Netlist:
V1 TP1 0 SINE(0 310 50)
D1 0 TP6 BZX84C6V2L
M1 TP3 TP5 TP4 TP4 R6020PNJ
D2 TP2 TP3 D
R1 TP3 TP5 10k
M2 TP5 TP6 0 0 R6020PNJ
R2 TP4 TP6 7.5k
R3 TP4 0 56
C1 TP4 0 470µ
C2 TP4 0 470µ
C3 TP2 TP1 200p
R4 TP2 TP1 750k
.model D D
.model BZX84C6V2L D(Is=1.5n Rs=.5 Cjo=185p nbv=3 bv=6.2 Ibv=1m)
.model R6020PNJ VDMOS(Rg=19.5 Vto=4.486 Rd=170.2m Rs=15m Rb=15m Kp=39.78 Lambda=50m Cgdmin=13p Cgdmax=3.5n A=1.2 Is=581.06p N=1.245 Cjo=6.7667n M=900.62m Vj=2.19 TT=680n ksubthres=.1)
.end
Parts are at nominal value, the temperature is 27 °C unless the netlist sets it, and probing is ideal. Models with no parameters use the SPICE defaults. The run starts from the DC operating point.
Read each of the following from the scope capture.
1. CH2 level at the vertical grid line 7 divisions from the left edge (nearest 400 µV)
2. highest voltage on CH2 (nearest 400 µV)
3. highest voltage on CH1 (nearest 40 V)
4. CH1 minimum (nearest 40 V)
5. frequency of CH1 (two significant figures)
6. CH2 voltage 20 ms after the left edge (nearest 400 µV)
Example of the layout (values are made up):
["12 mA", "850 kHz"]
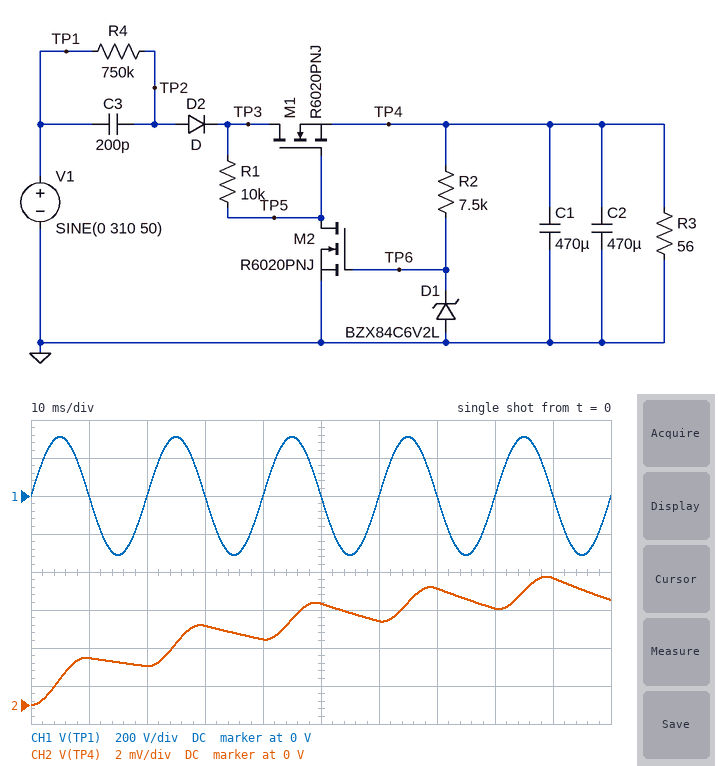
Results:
["6.0 mV", "6.8 mV", "320 V", "-320 V", "50 Hz", "2.0 mV"]
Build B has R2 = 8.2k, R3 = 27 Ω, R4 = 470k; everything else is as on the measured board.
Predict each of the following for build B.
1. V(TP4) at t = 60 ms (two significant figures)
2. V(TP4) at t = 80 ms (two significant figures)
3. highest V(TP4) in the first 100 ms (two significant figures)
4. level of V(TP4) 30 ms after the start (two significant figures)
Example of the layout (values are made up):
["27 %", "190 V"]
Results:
["4.0 mV", "4.2 mV", "6.6 mV", "5.2 mV"]
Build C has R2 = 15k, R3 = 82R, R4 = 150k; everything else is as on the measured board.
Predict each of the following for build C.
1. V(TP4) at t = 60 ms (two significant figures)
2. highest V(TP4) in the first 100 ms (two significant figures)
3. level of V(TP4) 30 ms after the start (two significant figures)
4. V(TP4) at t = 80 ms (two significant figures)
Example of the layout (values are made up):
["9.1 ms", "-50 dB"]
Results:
["27 mV", "41 mV", "23 mV", "32 mV"]
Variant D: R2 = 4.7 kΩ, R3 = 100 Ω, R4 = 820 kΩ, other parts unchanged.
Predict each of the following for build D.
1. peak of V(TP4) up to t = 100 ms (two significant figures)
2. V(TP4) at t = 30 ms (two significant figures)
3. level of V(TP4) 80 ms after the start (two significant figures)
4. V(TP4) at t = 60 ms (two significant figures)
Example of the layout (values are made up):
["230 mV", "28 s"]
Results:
["8.1 mV", "4.3 mV", "6.4 mV", "5.2 mV"]
